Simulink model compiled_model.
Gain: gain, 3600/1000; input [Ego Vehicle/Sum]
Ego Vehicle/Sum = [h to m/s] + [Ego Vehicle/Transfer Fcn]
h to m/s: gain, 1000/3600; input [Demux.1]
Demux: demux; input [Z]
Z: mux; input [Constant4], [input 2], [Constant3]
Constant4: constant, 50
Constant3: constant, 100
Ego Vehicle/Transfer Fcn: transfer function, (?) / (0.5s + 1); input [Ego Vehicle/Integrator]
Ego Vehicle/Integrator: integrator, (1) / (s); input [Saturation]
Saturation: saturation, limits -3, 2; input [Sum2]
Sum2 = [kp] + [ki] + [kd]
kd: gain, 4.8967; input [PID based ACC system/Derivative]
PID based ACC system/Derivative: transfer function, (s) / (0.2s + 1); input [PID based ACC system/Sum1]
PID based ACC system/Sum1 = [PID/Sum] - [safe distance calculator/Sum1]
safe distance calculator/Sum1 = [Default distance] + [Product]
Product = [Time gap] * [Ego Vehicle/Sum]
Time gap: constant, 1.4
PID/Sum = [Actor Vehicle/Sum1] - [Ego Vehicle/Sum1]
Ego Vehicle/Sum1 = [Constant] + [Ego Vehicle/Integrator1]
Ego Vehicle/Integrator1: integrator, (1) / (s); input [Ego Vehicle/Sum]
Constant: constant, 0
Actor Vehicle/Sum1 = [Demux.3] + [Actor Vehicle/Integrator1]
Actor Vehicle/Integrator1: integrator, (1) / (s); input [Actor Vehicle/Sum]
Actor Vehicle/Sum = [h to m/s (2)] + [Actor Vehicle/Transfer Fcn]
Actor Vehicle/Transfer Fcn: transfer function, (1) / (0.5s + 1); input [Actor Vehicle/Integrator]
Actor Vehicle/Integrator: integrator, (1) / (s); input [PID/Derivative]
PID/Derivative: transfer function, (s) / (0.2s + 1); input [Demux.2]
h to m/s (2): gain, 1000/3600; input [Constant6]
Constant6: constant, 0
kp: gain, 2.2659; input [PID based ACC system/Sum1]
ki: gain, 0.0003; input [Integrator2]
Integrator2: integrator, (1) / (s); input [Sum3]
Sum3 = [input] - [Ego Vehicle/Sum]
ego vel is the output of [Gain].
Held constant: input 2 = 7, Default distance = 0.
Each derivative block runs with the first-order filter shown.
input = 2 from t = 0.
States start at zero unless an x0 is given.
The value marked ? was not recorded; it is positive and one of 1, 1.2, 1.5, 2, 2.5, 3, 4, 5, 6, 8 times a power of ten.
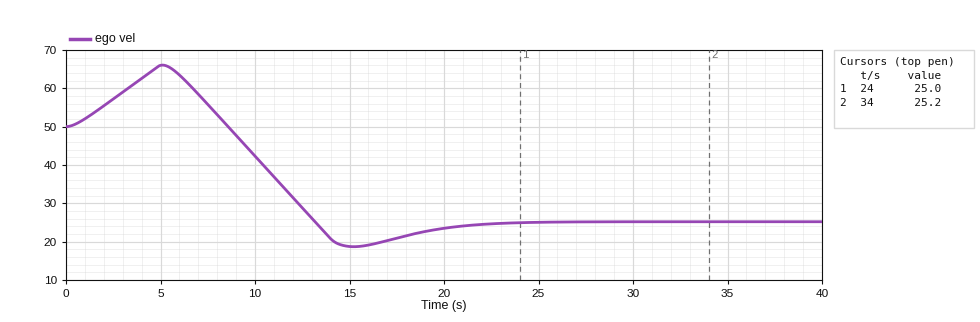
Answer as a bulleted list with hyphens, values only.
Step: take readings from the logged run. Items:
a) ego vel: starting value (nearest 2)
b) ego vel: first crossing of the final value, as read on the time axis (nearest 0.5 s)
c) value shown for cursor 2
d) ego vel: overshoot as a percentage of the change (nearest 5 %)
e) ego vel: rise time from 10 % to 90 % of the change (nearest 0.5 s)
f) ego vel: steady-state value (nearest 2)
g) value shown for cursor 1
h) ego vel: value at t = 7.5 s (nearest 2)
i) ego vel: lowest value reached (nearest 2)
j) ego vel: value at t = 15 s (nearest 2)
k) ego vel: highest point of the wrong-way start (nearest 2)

- 50
- 13.0 s
- 25.2
- 25 %
- 3.5 s
- 26
- 25.0
- 56
- 18
- 18
- 66
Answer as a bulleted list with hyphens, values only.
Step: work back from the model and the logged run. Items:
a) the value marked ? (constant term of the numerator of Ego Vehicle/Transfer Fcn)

- 0.5
